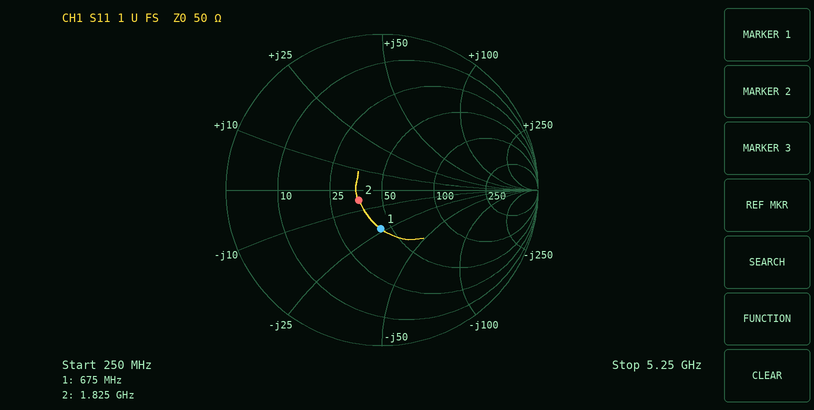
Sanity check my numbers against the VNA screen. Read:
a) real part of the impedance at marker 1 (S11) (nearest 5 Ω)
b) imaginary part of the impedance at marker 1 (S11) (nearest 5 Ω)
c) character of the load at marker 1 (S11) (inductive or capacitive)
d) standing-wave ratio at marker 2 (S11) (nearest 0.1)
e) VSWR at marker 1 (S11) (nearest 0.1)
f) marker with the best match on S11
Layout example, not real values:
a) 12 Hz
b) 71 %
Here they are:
a) 45 Ω
b) -25 Ω
c) capacitive
d) 1.4
e) 1.7
f) marker 2
